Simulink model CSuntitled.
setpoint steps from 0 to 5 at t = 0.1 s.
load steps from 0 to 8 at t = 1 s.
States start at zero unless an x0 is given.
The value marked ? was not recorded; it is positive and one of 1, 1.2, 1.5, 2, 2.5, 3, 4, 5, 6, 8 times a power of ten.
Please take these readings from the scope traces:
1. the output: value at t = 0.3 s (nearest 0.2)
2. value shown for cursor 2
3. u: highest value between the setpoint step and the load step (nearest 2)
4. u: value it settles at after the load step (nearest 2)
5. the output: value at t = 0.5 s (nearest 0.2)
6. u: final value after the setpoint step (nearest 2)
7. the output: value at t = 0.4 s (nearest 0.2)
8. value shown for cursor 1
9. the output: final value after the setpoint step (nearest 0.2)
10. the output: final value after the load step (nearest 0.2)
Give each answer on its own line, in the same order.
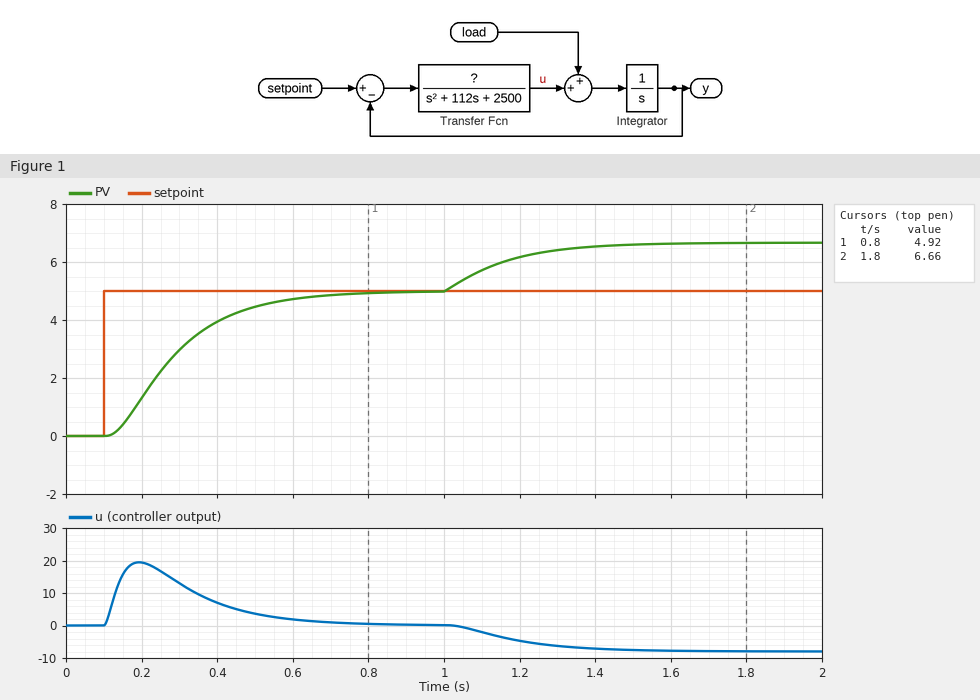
3.0
6.66
20
-8
4.4
0
4.0
4.92
5.0
6.6
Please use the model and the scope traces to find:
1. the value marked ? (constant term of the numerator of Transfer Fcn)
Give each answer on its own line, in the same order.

12000
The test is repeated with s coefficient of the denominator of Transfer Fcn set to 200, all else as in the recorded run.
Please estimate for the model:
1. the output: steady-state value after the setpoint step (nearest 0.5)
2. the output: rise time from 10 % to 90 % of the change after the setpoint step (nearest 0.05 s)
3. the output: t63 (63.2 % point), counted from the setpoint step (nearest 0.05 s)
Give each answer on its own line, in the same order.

5.0
0.30 s
0.25 s
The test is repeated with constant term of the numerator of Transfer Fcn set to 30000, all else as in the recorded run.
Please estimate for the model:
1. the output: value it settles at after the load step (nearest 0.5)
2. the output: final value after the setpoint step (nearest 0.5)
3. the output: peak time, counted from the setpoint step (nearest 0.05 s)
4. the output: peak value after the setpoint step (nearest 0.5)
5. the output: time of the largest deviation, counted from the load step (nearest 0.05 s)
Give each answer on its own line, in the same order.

5.5
5.0
0.25 s
5.5
0.20 s
